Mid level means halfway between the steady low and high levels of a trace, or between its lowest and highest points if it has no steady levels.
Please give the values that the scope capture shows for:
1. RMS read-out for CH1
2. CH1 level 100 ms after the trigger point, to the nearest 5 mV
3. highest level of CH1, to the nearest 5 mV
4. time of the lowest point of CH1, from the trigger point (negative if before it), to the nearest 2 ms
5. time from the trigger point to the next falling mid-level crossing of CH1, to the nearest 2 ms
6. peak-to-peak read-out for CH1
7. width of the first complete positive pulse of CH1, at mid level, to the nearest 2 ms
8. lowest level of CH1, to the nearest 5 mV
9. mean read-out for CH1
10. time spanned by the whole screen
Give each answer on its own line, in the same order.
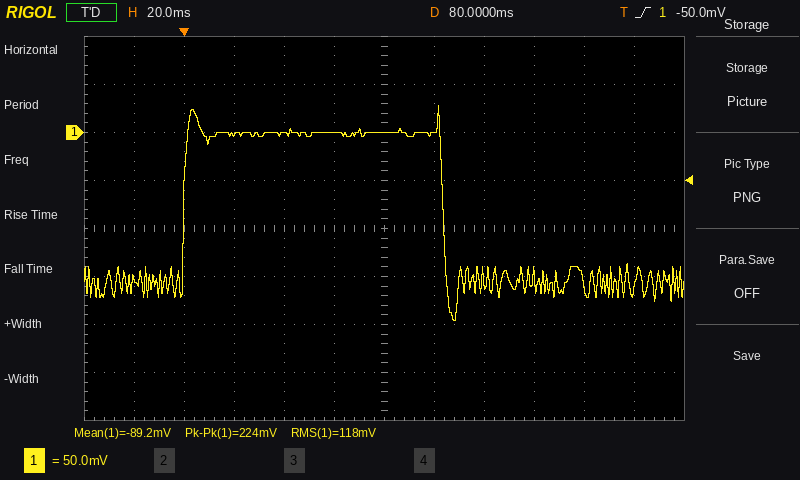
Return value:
118 mV
0 mV
30 mV
+108 ms
104 ms
224 mV
104 ms
-195 mV
-89.2 mV
240 ms
